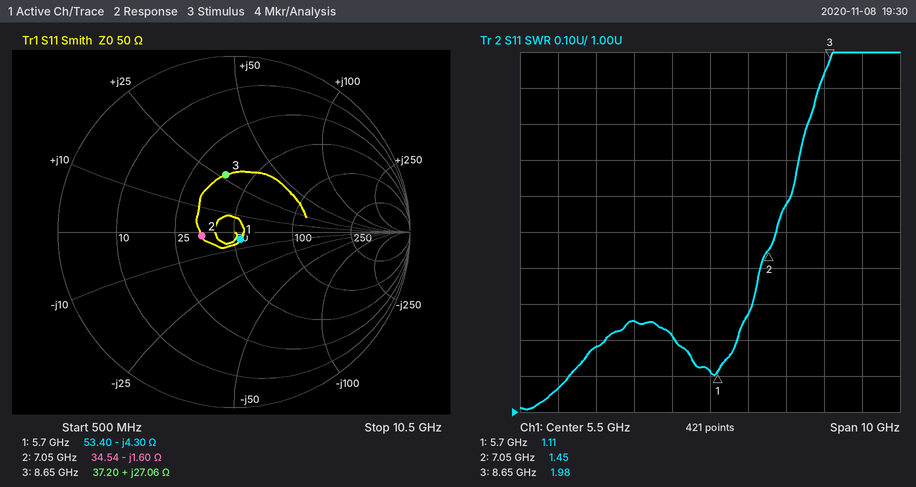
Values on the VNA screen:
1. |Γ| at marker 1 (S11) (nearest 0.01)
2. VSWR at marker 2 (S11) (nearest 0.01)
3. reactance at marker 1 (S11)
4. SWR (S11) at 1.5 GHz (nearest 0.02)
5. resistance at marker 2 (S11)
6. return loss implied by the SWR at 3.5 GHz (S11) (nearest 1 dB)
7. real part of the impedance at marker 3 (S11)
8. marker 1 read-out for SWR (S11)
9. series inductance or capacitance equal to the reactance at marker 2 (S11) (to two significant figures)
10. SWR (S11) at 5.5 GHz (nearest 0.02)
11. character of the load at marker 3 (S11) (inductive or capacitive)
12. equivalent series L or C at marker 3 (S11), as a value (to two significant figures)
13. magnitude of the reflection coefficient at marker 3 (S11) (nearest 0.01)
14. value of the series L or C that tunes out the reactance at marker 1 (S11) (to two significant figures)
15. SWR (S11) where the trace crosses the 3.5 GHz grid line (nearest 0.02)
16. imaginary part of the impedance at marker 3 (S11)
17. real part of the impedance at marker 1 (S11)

0.05
1.45
-4.30 Ω
1.06
34.54 Ω
19 dB
37.20 Ω
1.11
14 pF
1.12
inductive
500 pH
0.33
120 pH
1.26
+27.06 Ω
53.40 Ω
